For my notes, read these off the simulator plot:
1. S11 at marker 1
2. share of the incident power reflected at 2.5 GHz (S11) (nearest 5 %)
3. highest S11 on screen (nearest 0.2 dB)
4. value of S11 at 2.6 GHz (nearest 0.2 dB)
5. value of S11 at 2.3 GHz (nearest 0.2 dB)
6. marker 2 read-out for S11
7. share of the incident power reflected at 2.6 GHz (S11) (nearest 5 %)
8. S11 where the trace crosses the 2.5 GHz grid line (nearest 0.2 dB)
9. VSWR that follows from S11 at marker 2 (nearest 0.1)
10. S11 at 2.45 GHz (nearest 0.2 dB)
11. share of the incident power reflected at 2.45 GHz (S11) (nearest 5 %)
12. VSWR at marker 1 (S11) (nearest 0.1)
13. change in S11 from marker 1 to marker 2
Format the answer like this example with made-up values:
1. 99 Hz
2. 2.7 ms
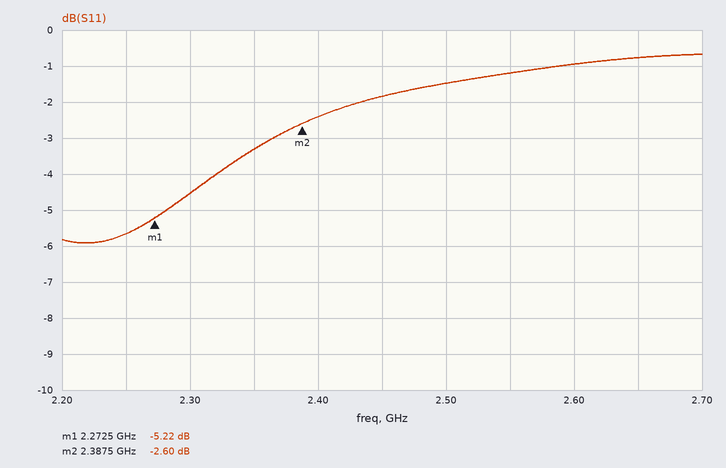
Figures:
1. -5.22 dB
2. 70 %
3. -0.6 dB
4. -1.0 dB
5. -4.6 dB
6. -2.60 dB
7. 80 %
8. -1.4 dB
9. 6.7
10. -1.8 dB
11. 65 %
12. 3.4
13. 2.62 dB
